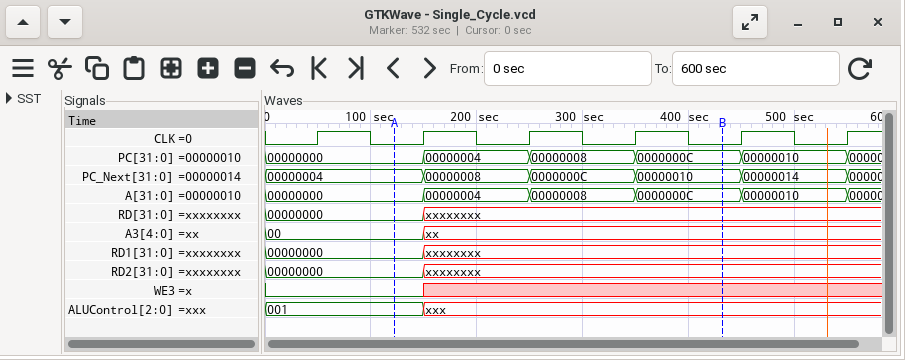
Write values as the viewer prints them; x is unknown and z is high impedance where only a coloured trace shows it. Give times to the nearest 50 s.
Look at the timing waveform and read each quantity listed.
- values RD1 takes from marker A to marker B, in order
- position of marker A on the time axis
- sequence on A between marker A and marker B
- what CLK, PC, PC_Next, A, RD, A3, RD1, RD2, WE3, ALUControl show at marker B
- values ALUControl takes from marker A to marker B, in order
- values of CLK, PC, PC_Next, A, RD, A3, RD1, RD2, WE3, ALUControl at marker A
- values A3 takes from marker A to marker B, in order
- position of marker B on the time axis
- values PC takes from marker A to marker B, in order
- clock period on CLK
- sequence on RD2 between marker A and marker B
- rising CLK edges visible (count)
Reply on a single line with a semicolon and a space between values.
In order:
00000000, xxxxxxxx; 100 s; 00000000, 00000004, 00000008, 0000000C; CLK=0, PC=0000000C, PC_Next=00000010, A=0000000C, RD=xxxxxxxx, A3=xx, RD1=xxxxxxxx, RD2=xxxxxxxx, WE3=x, ALUControl=xxx; 001, xxx; CLK=0, PC=00000000, PC_Next=00000004, A=00000000, RD=00000000, A3=00, RD1=00000000, RD2=00000000, WE3=0, ALUControl=001; 00, xx; 450 s; 00000000, 00000004, 00000008, 0000000C; 100 s; 00000000, xxxxxxxx; 6
